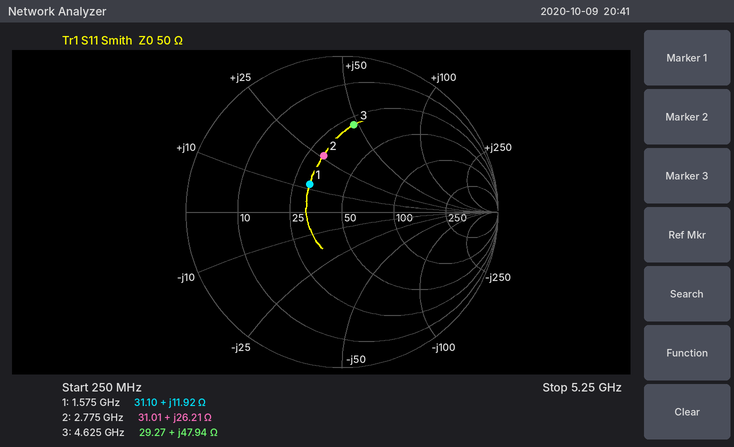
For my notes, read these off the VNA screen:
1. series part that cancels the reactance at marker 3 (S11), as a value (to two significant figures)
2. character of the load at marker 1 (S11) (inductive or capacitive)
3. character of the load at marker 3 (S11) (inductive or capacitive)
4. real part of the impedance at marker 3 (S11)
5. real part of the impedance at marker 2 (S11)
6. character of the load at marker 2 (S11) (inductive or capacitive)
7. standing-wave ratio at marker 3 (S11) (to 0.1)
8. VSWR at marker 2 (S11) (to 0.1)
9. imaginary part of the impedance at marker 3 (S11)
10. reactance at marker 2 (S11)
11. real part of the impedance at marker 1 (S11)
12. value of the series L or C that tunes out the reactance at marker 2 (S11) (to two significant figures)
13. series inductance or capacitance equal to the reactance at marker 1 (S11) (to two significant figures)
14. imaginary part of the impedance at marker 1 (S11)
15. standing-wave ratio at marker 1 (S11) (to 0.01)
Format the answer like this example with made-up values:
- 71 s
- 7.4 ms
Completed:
- 720 fF
- inductive
- inductive
- 29.27 Ω
- 31.01 Ω
- inductive
- 3.6
- 2.2
- +47.94 Ω
- +26.21 Ω
- 31.10 Ω
- 2.2 pF
- 1.2 nH
- +11.92 Ω
- 1.75
